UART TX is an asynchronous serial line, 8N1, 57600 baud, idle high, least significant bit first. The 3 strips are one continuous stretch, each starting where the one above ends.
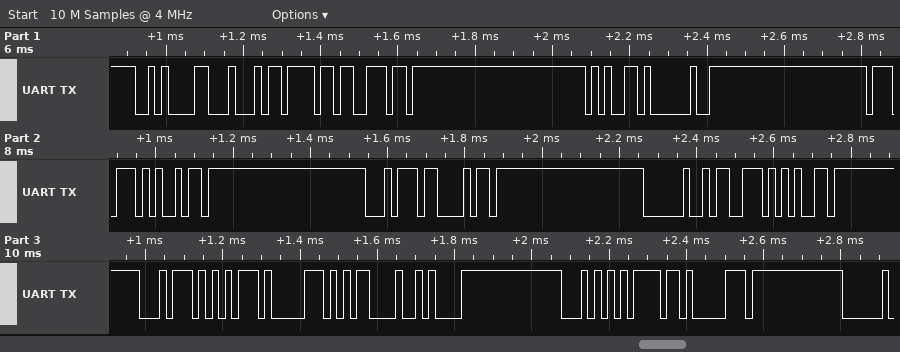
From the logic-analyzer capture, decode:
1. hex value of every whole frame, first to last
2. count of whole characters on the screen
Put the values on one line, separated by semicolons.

0x0A 0x44 0x6F 0x6E 0x65 0x20 0x77 0x69 0x74 0x68 0x20 0x73 0x65 0x74 0x75 0x70 0x0D 0x0A 0x54 0x6F 0x70; 21
